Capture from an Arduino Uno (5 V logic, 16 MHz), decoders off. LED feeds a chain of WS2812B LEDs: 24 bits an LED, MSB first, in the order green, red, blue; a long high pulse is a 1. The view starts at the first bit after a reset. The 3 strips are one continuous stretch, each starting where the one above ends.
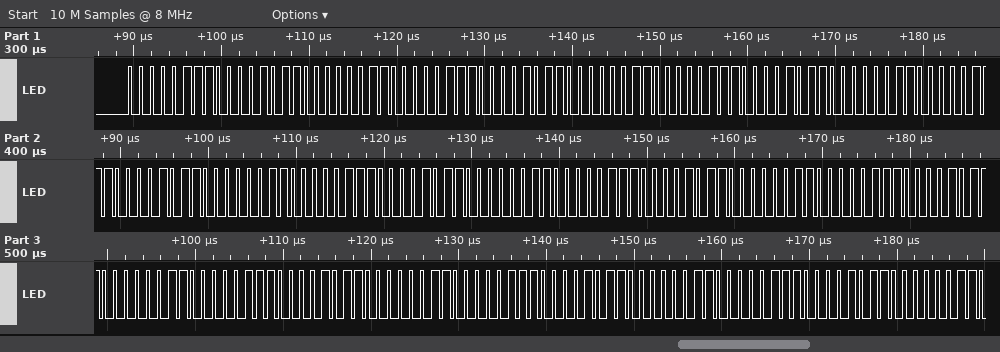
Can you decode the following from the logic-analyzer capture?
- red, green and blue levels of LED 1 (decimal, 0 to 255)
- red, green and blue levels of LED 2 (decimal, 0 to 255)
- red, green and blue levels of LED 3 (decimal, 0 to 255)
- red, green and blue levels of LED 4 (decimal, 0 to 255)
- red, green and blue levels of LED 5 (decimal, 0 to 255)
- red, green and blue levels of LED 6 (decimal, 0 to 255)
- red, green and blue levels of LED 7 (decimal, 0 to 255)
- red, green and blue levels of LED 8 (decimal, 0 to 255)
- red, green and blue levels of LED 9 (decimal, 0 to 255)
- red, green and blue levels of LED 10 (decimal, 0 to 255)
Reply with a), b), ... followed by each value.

a) 11, 7, 3
b) 11, 7, 3
c) 11, 7, 3
d) 11, 7, 3
e) 11, 7, 3
f) 11, 7, 3
g) 11, 7, 3
h) 11, 7, 3
i) 11, 7, 3
j) 11, 7, 3
